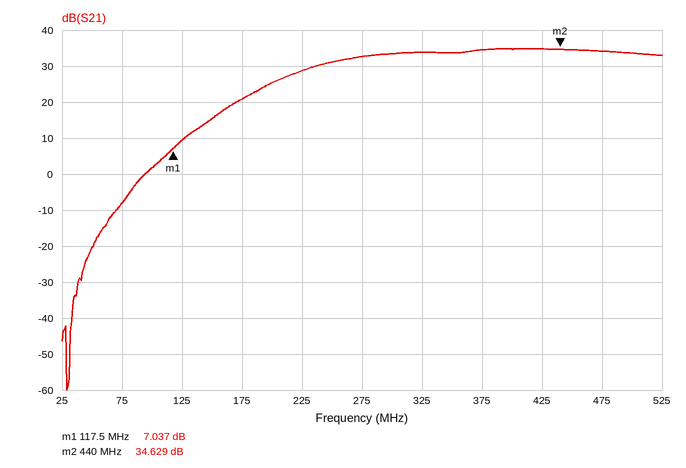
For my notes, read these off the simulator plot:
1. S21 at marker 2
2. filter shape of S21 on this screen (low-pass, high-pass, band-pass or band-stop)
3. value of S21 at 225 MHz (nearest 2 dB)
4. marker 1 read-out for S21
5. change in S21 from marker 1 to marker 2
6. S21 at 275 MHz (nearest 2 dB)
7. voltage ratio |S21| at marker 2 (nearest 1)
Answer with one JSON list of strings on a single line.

["34.629 dB", "high-pass", "28 dB", "7.037 dB", "27.592 dB", "32 dB", "54"]
